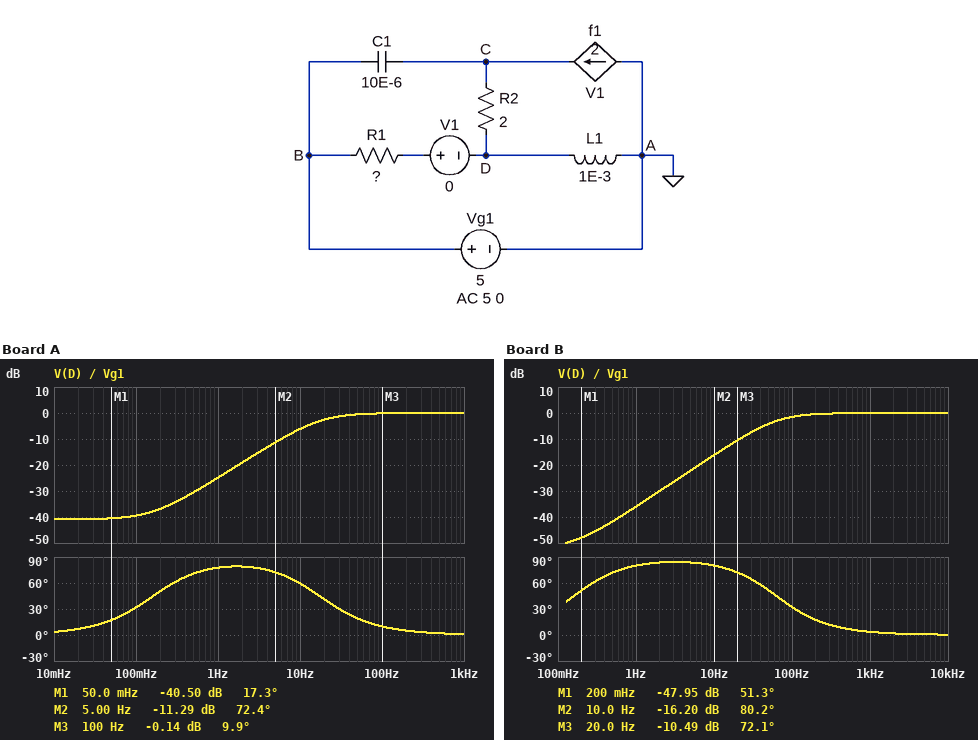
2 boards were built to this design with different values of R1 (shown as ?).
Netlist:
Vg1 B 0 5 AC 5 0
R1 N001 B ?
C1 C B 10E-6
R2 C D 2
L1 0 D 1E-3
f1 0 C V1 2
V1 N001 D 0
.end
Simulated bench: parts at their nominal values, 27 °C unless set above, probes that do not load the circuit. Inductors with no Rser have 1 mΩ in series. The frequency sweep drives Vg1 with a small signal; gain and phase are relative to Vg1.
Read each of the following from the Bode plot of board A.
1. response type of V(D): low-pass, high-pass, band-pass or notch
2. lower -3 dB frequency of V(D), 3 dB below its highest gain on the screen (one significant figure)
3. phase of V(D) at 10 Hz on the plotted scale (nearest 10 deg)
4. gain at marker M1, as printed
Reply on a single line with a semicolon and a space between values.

high-pass; 20 Hz; 60 deg; -40.50 dB
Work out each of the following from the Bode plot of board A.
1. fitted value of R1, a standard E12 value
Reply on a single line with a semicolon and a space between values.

0.33 Ω
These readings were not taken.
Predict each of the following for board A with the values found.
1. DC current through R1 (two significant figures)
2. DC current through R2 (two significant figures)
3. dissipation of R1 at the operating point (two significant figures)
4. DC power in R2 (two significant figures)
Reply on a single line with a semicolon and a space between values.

15 A; 30 A; 74 W; 1.8 kW
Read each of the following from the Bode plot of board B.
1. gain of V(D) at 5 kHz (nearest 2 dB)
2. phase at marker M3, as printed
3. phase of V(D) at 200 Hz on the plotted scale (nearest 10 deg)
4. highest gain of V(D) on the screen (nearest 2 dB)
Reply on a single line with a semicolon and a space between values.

0 dB; 72.1 deg; 20 deg; 0 dB
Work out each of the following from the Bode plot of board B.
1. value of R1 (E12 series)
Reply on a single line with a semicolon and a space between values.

1.2 Ω
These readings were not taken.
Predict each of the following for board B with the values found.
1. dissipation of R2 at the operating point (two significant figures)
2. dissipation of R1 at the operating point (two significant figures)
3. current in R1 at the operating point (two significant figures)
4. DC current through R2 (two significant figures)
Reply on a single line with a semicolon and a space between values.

140 W; 21 W; 4.2 A; 8.3 A
